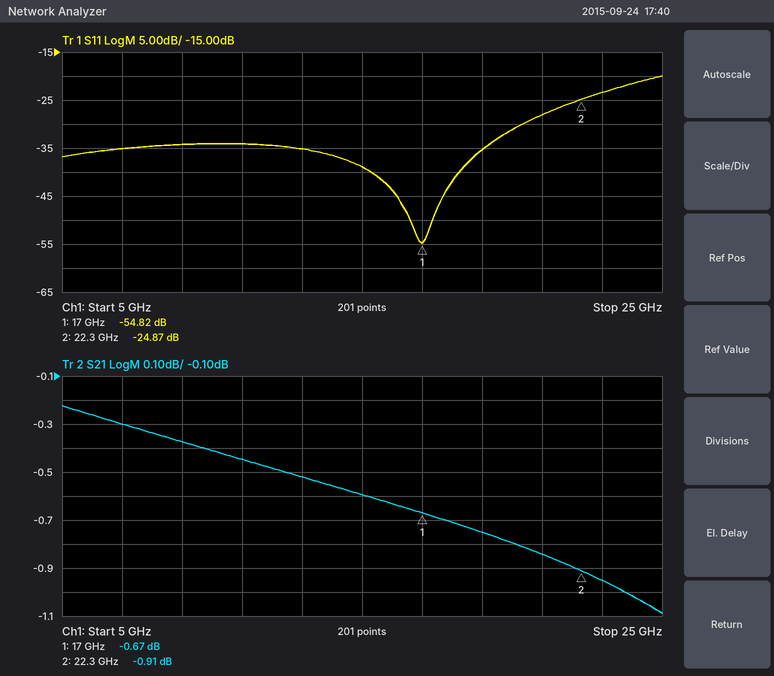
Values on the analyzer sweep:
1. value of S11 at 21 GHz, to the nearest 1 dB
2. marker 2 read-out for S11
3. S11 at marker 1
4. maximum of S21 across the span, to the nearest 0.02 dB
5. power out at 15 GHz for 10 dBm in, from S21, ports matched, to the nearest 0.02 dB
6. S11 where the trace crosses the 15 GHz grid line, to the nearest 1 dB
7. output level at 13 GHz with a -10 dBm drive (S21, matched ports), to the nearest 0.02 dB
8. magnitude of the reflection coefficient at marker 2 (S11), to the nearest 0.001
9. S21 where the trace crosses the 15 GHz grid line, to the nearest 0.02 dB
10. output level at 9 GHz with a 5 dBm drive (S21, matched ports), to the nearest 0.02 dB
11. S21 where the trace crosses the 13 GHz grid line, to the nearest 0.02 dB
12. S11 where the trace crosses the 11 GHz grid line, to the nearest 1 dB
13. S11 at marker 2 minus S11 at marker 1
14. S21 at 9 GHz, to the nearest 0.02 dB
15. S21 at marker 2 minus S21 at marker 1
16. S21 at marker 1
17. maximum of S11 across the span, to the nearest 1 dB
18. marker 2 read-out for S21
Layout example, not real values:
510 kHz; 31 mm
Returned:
-28 dB; -24.87 dB; -54.82 dB; -0.22 dB; 9.40 dBm; -39 dB; -10.52 dBm; 0.057; -0.60 dB; 4.62 dBm; -0.52 dB; -34 dB; 29.95 dB; -0.38 dB; -0.24 dB; -0.67 dB; -20 dB; -0.91 dB
